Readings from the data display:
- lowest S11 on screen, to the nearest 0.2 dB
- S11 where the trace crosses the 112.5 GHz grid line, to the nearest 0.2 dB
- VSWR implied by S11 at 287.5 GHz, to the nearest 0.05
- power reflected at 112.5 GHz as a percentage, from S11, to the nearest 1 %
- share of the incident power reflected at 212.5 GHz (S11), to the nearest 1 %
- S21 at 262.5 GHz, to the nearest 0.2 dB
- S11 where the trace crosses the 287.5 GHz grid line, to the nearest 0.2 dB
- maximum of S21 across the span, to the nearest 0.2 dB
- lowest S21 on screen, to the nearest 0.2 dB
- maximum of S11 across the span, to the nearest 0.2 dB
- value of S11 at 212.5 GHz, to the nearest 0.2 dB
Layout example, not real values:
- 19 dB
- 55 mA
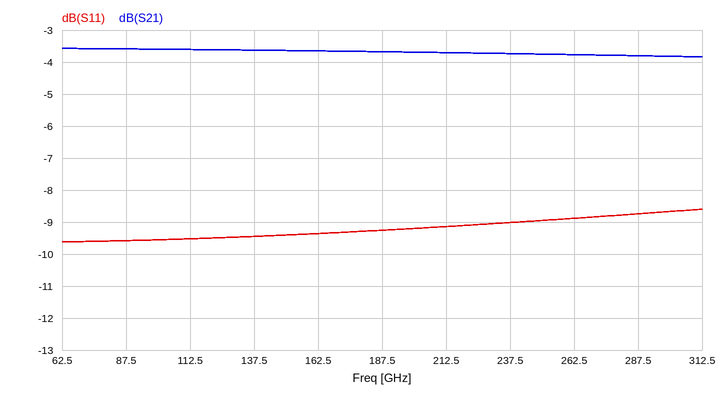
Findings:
- -9.6 dB
- -9.6 dB
- 2.15
- 11 %
- 12 %
- -3.8 dB
- -8.8 dB
- -3.6 dB
- -3.8 dB
- -8.6 dB
- -9.2 dB
